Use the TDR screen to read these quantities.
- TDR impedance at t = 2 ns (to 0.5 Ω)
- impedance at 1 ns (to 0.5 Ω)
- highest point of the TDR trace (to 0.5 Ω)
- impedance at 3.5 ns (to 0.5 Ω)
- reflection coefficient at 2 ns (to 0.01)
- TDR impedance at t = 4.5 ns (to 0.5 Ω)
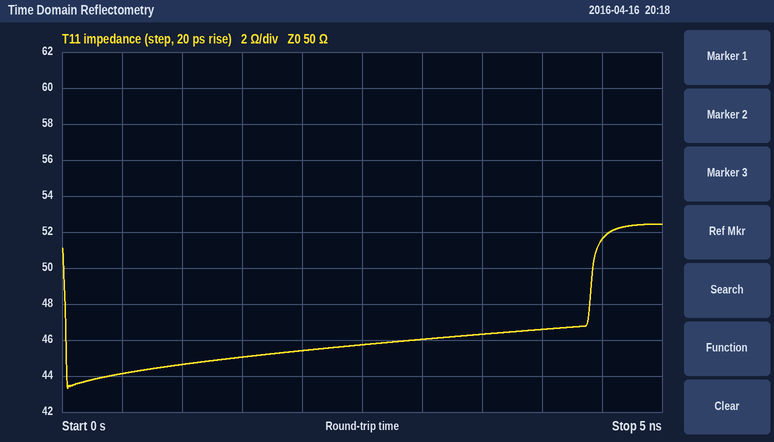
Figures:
45.5 Ω
44.5 Ω
52.5 Ω
46.5 Ω
-0.05
51.5 Ω
